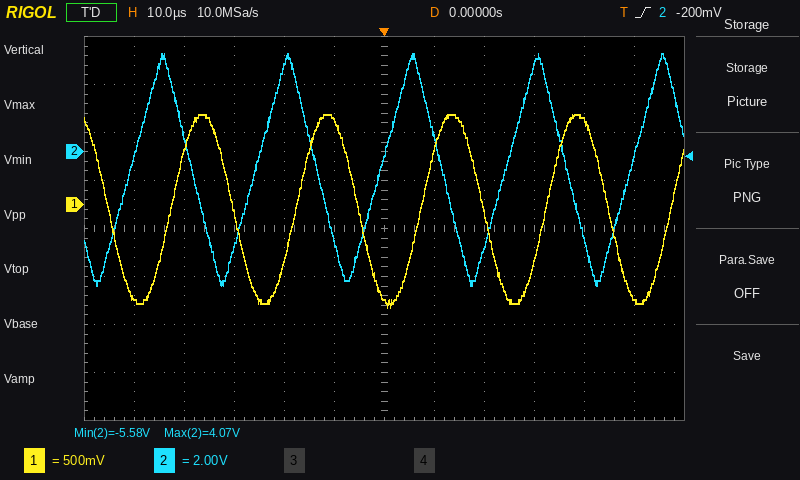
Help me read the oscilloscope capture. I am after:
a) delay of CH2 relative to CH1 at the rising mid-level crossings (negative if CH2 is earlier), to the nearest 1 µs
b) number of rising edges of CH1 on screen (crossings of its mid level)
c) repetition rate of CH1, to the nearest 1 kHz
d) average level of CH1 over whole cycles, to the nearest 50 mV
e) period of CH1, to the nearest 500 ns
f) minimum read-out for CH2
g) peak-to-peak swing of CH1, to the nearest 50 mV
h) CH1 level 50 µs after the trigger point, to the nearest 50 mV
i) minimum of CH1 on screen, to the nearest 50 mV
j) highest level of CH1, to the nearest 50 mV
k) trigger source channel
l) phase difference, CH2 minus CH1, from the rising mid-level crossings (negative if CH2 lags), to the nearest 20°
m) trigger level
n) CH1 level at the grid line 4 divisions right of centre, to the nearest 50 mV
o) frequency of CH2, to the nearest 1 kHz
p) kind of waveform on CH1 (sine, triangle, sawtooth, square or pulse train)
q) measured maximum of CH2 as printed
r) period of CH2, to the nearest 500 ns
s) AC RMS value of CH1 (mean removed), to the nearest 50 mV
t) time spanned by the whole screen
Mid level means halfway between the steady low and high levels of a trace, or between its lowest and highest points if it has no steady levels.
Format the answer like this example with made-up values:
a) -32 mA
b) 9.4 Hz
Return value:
a) -8 µs
b) 5
c) 40 kHz
d) -50 mV
e) 25.0 µs
f) -5.58 V
g) 2.00 V
h) -1.00 V
i) -1.05 V
j) 950 mV
k) CH2
l) +120°
m) -200 mV
n) 850 mV
o) 40 kHz
p) sine
q) 4.07 V
r) 25.0 µs
s) 700 mV
t) 120 µs
